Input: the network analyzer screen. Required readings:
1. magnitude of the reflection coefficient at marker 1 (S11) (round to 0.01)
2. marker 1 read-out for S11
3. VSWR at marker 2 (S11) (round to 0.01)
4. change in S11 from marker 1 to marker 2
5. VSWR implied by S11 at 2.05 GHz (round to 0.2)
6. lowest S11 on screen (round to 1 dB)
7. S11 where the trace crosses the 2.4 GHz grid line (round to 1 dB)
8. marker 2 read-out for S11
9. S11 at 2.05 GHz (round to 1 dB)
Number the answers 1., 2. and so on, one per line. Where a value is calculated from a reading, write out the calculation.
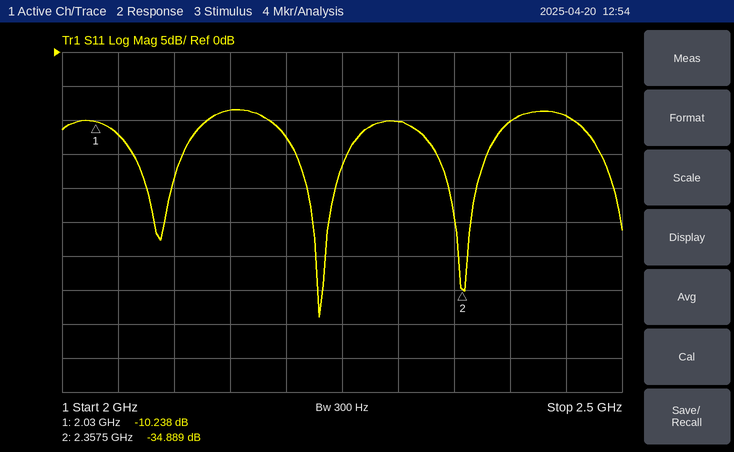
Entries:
1. 10^(-10.238/20) ≈ 0.31
2. -10.238 dB
3. (1 + 0.0180)/(1 − 0.0180) ≈ 1.04
4. -34.889 − (-10.238) = -24.651 dB
5. |Γ| = 10^(-12/20) = 0.2512; VSWR = (1 + 0.2512)/(1 − 0.2512) ≈ 1.67, so 1.6 to the nearest 0.2
6. -39 dB
7. -10 dB
8. -34.889 dB
9. -12 dB
